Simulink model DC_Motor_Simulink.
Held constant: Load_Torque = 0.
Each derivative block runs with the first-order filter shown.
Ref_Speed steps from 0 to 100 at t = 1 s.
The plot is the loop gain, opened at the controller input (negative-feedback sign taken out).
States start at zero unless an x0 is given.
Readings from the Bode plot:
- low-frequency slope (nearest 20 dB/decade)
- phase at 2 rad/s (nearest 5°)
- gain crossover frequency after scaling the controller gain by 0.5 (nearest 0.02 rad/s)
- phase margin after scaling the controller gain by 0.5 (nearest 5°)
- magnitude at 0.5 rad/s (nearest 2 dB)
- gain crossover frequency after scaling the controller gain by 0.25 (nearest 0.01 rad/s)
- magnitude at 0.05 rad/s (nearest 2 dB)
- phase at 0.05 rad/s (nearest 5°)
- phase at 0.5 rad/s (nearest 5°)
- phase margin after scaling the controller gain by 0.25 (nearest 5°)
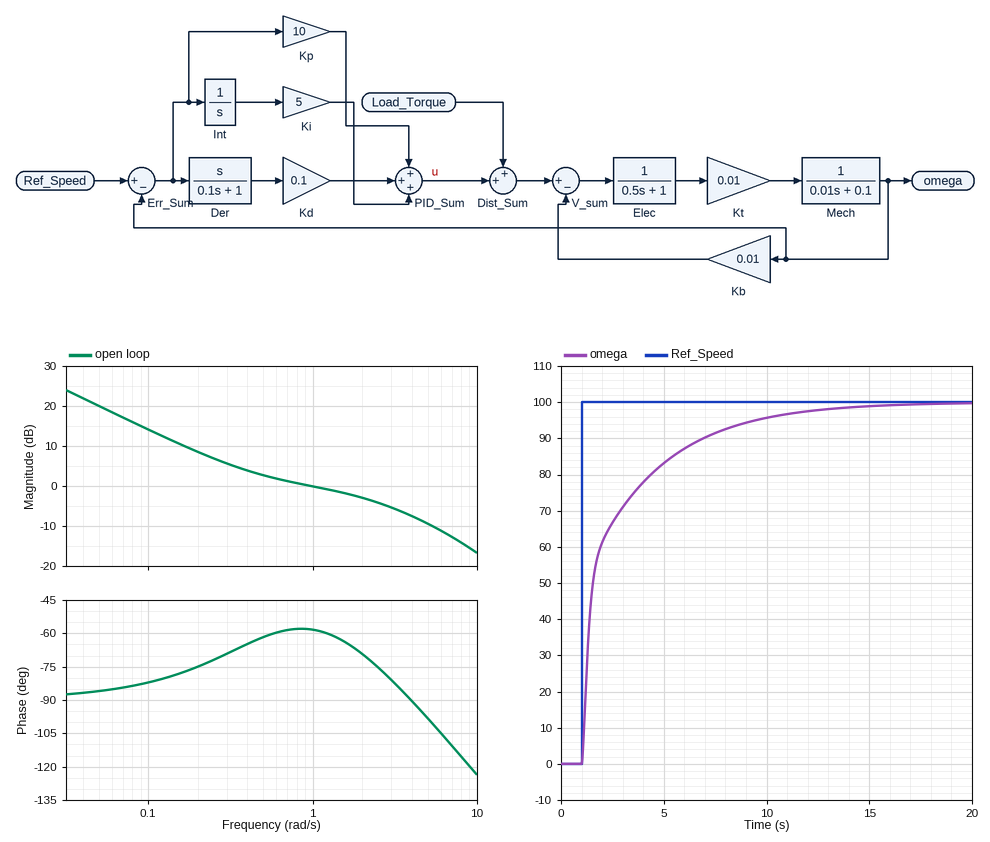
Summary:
-20 dB/decade
-70°
0.28 rad/s
110°
2 dB
0.13 rad/s
20 dB
-85°
-60°
100°
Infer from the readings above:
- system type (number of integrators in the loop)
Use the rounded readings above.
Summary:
1
